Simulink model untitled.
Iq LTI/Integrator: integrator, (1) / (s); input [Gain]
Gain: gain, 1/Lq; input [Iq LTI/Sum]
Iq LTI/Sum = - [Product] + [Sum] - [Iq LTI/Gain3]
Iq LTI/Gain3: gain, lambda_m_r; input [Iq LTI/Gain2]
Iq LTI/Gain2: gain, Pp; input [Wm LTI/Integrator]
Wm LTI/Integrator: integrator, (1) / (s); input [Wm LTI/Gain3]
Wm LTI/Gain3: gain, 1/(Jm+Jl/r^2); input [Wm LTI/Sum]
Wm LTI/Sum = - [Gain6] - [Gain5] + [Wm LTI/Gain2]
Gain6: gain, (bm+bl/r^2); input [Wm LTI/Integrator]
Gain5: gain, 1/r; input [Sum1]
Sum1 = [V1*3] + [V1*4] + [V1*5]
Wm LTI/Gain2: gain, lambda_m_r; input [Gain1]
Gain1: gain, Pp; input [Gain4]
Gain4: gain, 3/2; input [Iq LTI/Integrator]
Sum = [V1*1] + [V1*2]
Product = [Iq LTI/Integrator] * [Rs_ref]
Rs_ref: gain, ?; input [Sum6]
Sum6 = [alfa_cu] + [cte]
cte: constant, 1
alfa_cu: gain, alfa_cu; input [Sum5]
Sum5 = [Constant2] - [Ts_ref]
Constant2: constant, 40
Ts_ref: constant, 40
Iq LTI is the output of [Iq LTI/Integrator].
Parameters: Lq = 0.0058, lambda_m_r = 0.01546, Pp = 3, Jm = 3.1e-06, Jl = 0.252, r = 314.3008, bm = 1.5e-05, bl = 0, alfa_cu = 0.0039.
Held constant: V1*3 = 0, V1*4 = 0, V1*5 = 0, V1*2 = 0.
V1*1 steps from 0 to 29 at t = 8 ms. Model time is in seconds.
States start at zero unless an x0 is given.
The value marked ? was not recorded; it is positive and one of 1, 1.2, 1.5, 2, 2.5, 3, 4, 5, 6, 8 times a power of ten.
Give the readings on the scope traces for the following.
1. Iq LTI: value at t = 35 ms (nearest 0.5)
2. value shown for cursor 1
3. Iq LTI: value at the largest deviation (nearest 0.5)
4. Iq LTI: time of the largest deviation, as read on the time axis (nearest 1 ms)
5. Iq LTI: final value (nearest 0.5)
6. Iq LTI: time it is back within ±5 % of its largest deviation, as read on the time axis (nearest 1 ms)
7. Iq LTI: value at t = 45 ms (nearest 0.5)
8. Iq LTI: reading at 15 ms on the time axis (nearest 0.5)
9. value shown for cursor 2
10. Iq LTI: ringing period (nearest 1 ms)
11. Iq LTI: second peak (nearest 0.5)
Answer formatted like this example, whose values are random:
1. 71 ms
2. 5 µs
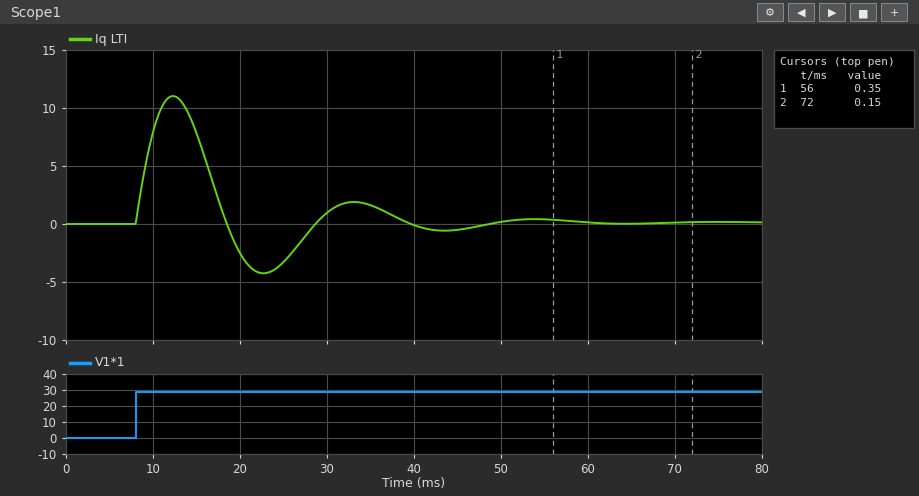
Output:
1. 1.5
2. 0.35
3. 11.0
4. 12 ms
5. 0.0
6. 46 ms
7. -0.5
8. 8.0
9. 0.15
10. 21 ms
11. 2.0
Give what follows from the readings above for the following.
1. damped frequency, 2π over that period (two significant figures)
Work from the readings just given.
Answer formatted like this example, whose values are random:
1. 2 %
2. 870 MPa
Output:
1. 0.30 rad/ms
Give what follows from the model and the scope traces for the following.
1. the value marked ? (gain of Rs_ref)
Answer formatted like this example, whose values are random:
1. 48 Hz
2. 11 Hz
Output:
1. 1
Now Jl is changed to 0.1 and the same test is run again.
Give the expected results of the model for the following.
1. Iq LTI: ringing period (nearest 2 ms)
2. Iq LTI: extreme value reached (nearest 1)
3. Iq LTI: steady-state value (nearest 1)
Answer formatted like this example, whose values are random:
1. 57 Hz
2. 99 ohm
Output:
1. 18 ms
2. 10
3. 0
